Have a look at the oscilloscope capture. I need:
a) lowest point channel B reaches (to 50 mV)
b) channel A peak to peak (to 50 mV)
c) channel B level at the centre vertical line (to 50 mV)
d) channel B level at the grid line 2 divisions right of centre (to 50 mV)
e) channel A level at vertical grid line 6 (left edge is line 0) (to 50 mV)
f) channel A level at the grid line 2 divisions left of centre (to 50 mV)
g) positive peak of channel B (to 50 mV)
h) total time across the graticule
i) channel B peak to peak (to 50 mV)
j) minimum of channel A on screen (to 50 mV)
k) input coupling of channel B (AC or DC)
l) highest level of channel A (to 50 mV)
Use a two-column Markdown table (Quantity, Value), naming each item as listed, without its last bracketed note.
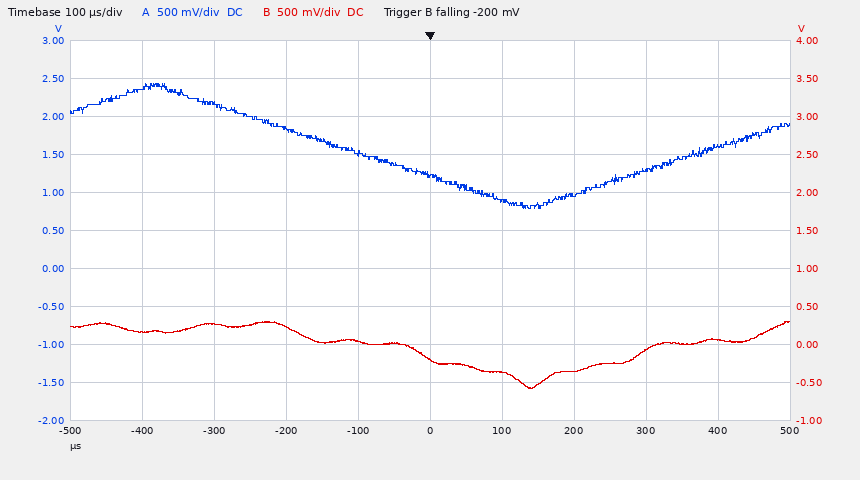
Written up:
| Quantity | Value |
|---|---|
| lowest point channel B reaches | -600 mV |
| channel A peak to peak | 1.65 V |
| channel B level at the centre vertical line | -200 mV |
| channel B level at the grid line 2 divisions right of centre | -350 mV |
| channel A level at vertical grid line 6 (left edge is line 0) | 900 mV |
| channel A level at the grid line 2 divisions left of centre | 1.85 V |
| positive peak of channel B | 300 mV |
| total time across the graticule | 1 ms |
| channel B peak to peak | 900 mV |
| minimum of channel A on screen | 800 mV |
| input coupling of channel B | DC |
| highest level of channel A | 2.45 V |
